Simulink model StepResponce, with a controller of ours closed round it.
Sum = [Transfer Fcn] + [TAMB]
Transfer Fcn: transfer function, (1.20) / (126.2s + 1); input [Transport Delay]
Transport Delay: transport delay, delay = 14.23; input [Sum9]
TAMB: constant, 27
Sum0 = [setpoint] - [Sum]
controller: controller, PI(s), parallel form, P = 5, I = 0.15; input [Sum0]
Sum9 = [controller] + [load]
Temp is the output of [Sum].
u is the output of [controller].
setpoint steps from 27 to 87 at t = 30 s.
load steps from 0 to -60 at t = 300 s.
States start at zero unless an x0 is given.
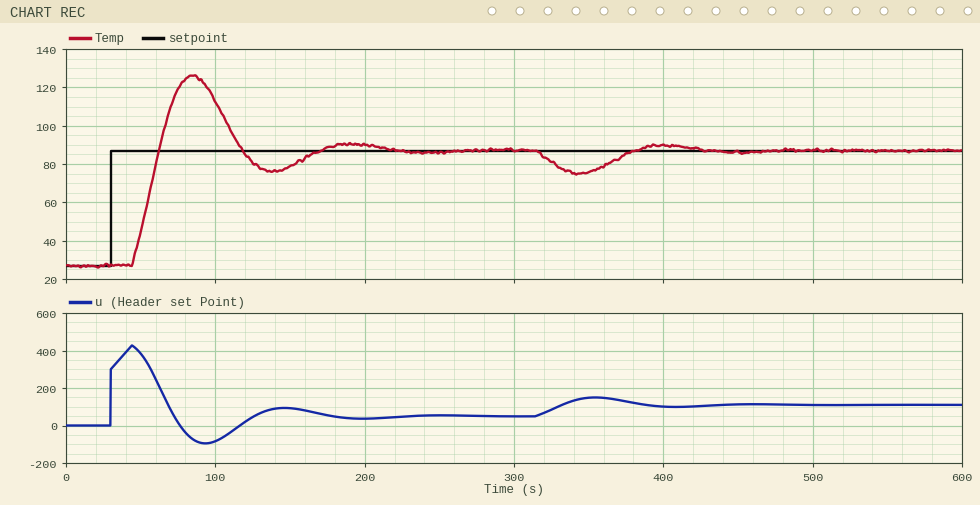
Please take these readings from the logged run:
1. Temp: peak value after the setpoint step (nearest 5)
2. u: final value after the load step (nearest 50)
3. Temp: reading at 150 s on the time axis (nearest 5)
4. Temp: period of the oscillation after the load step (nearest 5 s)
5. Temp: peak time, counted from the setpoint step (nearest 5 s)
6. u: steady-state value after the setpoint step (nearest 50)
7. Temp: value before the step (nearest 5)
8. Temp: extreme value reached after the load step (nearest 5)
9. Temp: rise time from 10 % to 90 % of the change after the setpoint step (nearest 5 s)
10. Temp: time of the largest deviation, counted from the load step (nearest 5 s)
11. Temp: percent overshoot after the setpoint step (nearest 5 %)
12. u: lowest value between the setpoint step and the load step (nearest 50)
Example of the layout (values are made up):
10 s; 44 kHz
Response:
125; 100; 80; 110 s; 55 s; 50; 25; 75; 15 s; 45 s; 65 %; -100
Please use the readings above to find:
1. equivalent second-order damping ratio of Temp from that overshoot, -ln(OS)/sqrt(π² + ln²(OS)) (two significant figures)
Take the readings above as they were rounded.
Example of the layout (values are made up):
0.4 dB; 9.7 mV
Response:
0.14
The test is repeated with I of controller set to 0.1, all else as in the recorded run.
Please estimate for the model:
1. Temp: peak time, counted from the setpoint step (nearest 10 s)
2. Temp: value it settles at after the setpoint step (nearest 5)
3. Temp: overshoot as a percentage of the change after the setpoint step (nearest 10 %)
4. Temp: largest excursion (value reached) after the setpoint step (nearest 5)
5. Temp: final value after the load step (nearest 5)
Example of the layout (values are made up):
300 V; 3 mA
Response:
50 s; 85; 40 %; 115; 85
